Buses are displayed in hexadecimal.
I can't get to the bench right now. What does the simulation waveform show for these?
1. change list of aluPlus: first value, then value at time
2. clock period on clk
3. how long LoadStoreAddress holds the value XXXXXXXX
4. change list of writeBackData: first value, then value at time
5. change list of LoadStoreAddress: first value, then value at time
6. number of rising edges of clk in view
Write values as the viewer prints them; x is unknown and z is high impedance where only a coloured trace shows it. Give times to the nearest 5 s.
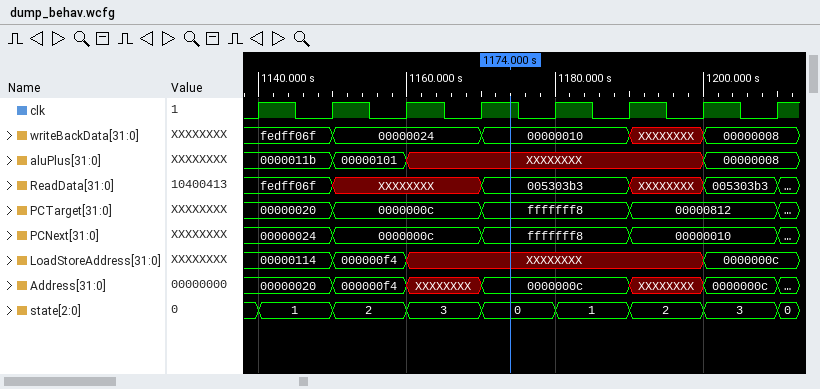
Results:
0000011b, 00000101 at 1150 s, XXXXXXXX at 1160 s, 00000008 at 1200 s
10 s
40 s
fedff06f, 00000024 at 1150 s, 00000010 at 1170 s, XXXXXXXX at 1190 s, 00000008 at 1200 s
00000114, 000000f4 at 1150 s, XXXXXXXX at 1160 s, 0000000c at 1200 s
8
